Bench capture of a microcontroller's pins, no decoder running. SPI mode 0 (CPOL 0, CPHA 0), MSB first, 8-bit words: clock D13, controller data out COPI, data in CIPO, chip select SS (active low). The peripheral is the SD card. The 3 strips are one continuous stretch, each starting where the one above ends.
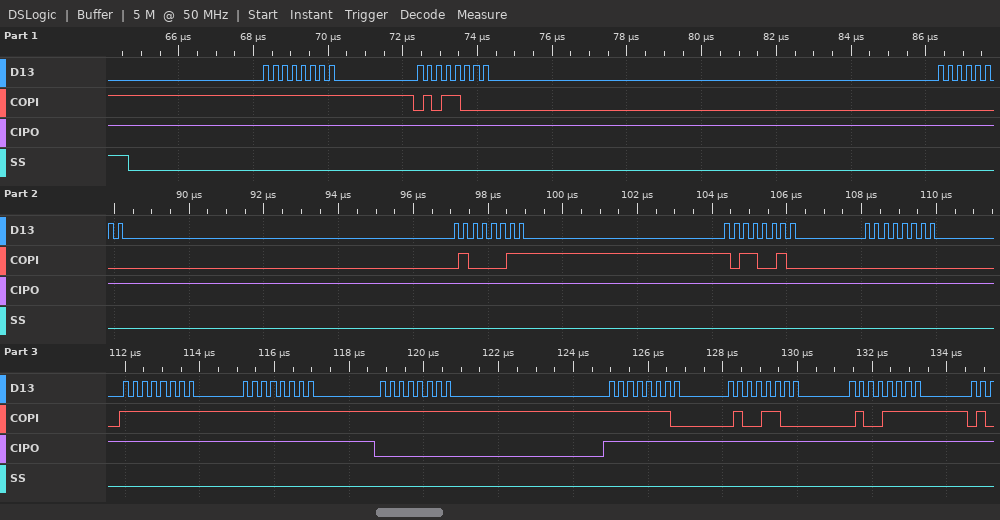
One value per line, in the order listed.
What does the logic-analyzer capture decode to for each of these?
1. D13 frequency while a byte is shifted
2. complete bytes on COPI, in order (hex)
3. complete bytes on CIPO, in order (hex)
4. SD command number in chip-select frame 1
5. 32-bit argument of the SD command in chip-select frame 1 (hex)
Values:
4 MHz
FF 58 00 43 B2 00 FF FF FF FE 4C 4F
FF FF FF FF FF FF FF FF 00 FF FF FF
CMD24
0x0043B200
